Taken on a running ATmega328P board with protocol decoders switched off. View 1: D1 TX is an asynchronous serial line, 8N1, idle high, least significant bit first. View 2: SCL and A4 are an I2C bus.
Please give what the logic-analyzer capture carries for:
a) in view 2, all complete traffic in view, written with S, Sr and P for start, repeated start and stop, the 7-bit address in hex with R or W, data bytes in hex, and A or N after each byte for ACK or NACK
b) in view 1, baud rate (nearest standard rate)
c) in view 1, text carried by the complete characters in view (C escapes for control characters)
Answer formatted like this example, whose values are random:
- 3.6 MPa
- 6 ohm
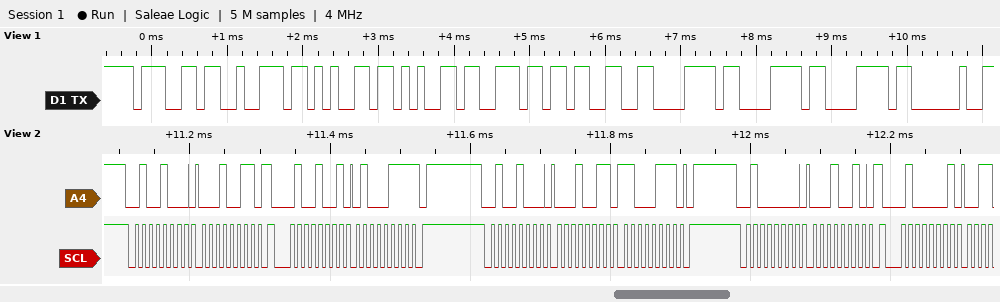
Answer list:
- S 24W A 13 A Sr 24R A 47 N P S 24W A 13 A C7 A P S 20W A 12 A Sr 20R A
- 9600 baud
- "green3xxx "
